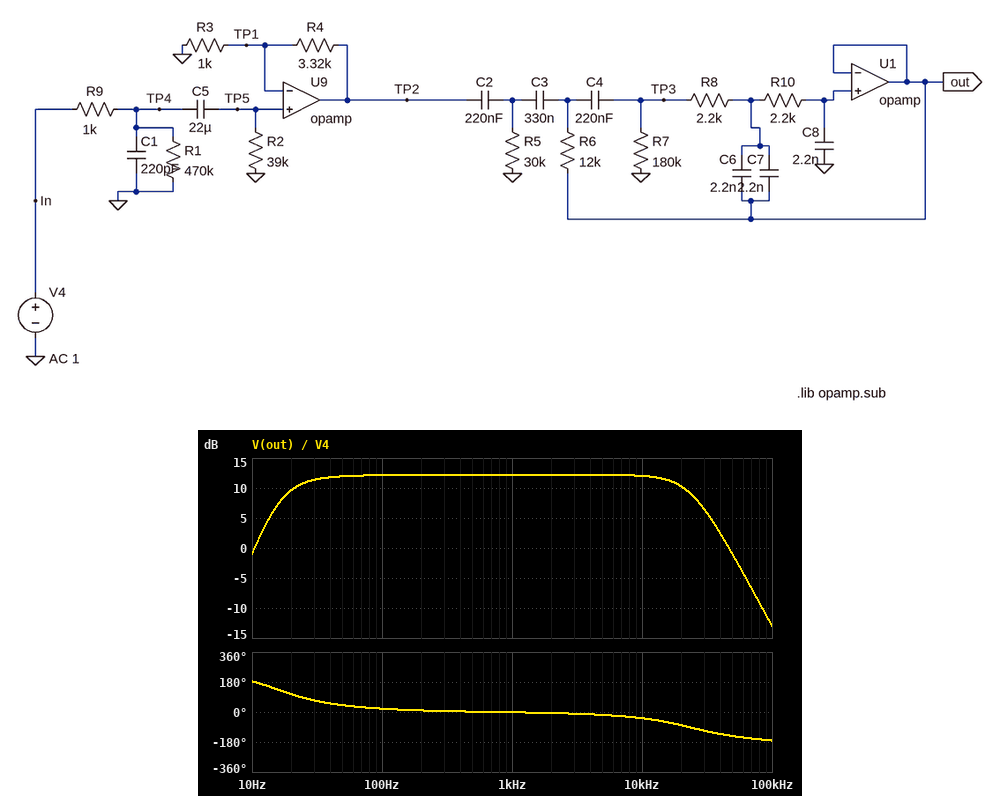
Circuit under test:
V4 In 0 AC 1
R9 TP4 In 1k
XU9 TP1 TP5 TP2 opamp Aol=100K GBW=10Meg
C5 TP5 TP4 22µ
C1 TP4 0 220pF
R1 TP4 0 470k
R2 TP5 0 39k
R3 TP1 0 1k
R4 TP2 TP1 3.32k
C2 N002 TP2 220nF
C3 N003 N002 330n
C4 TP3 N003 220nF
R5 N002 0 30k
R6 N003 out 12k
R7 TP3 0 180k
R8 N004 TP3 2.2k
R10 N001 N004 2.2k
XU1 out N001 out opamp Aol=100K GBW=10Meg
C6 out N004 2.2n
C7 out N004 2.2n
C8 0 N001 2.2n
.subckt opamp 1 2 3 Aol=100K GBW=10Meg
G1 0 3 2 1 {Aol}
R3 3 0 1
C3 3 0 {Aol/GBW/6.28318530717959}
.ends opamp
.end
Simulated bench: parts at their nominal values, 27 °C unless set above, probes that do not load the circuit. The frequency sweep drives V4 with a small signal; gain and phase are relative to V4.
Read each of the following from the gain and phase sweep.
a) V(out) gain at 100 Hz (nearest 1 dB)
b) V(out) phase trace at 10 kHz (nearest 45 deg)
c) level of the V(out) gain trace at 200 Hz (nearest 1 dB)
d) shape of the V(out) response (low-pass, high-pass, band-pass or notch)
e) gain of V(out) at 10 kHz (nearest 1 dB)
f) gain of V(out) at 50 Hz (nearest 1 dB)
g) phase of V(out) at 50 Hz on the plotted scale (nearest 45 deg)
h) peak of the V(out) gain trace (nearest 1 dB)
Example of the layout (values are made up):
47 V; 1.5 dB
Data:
12 dB; -45 deg; 12 dB; band-pass; 12 dB; 12 dB; 45 deg; 12 dB
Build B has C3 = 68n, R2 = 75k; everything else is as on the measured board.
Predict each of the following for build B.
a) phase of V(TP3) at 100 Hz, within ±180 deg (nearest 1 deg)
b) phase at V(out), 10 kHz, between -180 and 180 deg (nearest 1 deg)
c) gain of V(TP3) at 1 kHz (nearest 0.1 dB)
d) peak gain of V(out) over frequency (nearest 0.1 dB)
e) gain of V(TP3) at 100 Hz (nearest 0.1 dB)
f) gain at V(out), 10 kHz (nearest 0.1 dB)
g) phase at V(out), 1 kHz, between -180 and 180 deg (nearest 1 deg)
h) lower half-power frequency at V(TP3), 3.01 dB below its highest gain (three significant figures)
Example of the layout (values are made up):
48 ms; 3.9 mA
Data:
27 deg; -37 deg; 12.0 dB; 13.1 dB; 12.3 dB; 11.8 dB; -1 deg; 26.6 Hz
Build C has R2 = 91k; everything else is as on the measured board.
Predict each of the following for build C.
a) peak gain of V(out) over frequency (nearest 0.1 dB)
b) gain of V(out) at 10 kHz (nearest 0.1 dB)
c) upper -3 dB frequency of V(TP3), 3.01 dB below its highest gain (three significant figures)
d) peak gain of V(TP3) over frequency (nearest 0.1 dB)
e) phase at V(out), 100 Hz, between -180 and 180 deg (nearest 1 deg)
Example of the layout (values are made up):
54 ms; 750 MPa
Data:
12.3 dB; 12.1 dB; 684 kHz; 12.5 dB; 20 deg
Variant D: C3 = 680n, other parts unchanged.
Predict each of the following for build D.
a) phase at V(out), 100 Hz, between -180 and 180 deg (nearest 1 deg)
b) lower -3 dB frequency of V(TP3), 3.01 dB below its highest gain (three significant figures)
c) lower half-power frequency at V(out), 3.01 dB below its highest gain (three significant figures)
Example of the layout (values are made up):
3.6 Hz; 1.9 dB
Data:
19 deg; 21.4 Hz; 20.8 Hz
